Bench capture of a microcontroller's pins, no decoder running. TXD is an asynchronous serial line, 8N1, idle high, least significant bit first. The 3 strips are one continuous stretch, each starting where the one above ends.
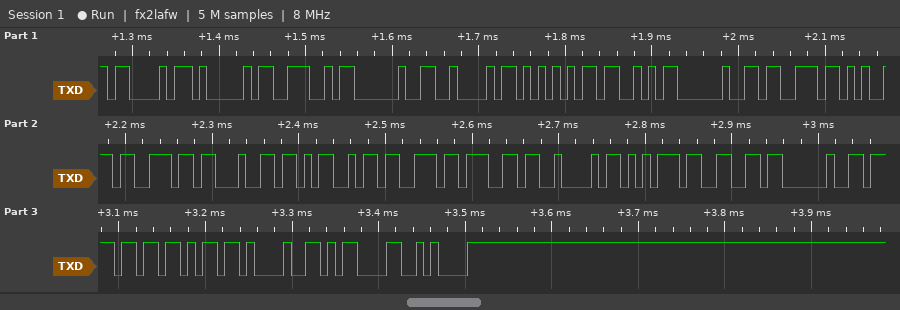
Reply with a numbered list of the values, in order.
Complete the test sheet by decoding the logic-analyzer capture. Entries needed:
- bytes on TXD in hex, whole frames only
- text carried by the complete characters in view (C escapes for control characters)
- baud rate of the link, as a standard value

1. 43 41 4E 20 42 55 53 20 73 65 6E 64 4D 73 67 42 75 66 20 6F 6B 21 0D 0A
2. "CAN BUS sendMsgBuf ok!\r\n"
3. 115200 baud
